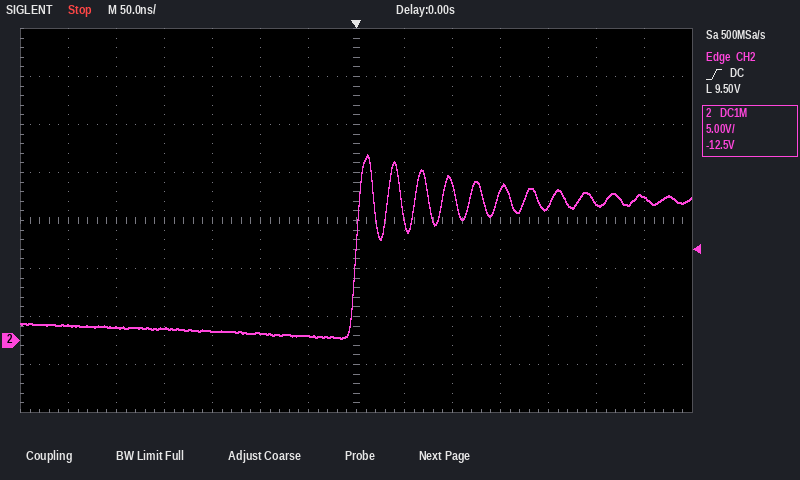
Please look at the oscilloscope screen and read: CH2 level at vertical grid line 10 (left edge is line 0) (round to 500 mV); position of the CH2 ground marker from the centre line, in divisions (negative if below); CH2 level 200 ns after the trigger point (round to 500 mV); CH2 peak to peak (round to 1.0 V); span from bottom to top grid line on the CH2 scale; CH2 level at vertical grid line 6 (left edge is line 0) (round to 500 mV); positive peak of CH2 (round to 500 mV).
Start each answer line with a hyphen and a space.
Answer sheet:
- 15.5 V
- -2.5 div
- 14.0 V
- 19.0 V
- 40 V
- 500 mV
- 19.5 V
